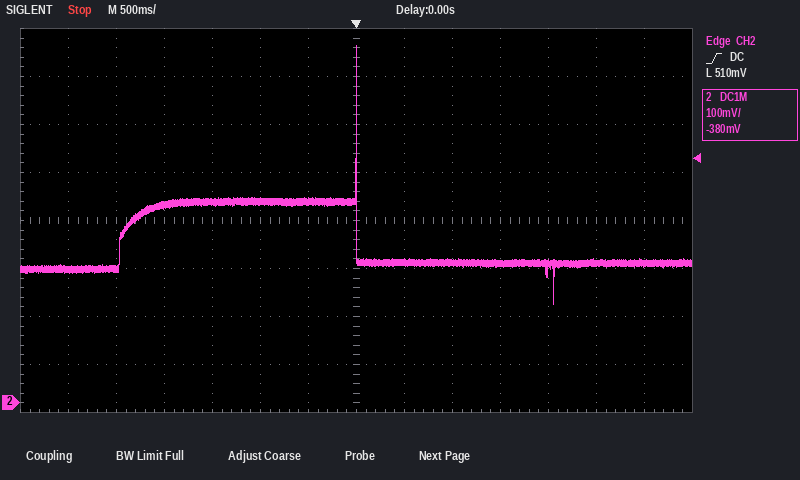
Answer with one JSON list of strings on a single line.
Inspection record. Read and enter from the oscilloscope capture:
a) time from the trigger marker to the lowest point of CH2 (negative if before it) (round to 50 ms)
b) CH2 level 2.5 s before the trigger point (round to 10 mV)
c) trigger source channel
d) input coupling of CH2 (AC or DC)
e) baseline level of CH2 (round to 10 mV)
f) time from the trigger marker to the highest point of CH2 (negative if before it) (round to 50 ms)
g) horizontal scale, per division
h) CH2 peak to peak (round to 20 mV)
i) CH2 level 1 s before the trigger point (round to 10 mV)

["+2.05 s", "280 mV", "CH2", "DC", "290 mV", "0 ms", "500 ms", "540 mV", "420 mV"]
